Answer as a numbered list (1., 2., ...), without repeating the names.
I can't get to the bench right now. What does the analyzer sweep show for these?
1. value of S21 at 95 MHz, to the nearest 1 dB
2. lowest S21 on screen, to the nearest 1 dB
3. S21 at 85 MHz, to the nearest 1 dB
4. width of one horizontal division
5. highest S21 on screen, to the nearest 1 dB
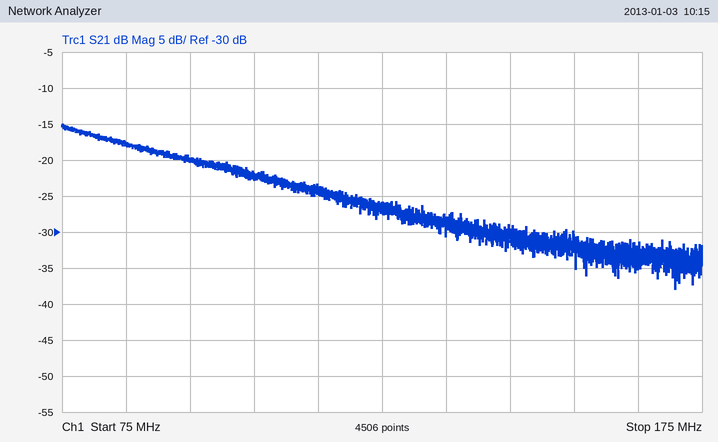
1. -20 dB
2. -38 dB
3. -18 dB
4. 10 MHz
5. -15 dB
